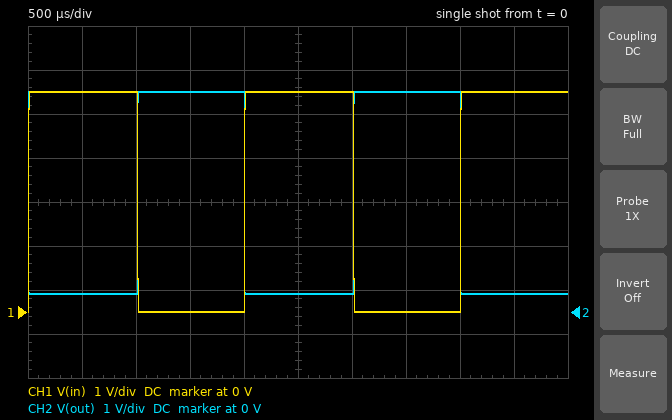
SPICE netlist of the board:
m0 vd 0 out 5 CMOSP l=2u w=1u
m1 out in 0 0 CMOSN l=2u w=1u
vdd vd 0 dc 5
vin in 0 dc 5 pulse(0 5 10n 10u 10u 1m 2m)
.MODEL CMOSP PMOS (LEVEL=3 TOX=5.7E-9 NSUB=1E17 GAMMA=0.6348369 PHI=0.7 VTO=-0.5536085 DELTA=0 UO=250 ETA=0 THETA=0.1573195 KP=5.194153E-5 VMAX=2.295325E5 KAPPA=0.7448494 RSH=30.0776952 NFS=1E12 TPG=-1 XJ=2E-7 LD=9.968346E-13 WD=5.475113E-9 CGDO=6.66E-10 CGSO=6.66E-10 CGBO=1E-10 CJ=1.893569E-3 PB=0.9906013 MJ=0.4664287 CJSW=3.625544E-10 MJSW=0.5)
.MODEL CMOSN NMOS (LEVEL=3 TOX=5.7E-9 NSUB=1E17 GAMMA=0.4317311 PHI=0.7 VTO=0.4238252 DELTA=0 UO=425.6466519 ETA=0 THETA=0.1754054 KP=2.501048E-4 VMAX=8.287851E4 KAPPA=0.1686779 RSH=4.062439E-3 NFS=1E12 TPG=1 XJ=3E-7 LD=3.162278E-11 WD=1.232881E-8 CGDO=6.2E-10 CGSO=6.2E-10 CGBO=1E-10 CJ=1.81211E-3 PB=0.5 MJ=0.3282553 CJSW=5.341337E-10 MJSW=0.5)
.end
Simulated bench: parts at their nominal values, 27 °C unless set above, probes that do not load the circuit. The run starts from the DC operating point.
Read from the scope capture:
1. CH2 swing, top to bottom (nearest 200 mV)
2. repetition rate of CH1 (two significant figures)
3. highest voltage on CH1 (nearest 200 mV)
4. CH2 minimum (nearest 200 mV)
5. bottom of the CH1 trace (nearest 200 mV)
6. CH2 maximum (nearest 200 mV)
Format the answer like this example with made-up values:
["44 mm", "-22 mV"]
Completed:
["4.6 V", "500 Hz", "5.0 V", "400 mV", "0 V", "5.0 V"]
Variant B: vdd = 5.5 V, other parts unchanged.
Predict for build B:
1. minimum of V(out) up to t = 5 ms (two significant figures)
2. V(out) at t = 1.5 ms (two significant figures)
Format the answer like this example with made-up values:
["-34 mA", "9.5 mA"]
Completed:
["490 mV", "5.5 V"]
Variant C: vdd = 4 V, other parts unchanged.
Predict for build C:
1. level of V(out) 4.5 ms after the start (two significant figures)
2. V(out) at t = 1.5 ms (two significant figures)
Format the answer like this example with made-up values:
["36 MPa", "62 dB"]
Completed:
["270 mV", "4.0 V"]
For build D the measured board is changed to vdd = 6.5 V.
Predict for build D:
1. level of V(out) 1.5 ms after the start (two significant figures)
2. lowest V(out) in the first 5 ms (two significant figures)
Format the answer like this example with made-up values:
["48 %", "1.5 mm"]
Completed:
["6.5 V", "670 mV"]
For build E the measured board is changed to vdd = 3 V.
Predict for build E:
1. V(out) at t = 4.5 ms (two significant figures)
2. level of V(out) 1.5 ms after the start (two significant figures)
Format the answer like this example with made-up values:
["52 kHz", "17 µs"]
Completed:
["150 mV", "3.0 V"]
